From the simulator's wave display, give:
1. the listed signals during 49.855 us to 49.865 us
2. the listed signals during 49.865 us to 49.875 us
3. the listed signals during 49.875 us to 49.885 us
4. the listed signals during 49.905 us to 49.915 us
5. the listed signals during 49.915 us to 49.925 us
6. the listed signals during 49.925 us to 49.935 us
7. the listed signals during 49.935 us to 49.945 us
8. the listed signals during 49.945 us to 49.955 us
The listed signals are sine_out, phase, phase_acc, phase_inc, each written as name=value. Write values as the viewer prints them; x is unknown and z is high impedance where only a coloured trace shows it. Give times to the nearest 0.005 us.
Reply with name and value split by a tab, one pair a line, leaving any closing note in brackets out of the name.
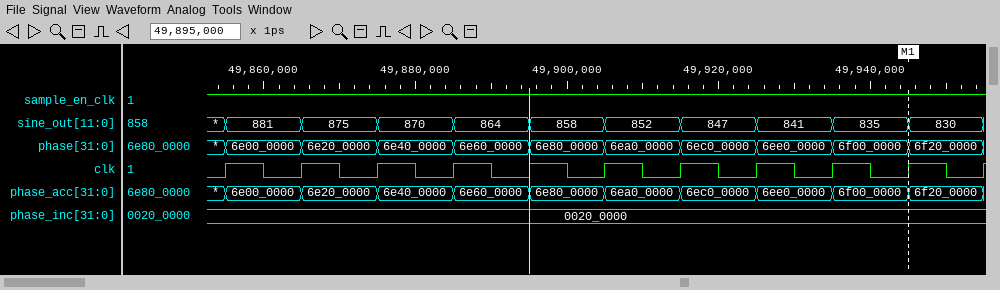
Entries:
the listed signals during 49.855 us to 49.865 us	sine_out=881, phase=6e00_0000, phase_acc=6e00_0000, phase_inc=0020_0000
the listed signals during 49.865 us to 49.875 us	sine_out=875, phase=6e20_0000, phase_acc=6e20_0000, phase_inc=0020_0000
the listed signals during 49.875 us to 49.885 us	sine_out=870, phase=6e40_0000, phase_acc=6e40_0000, phase_inc=0020_0000
the listed signals during 49.905 us to 49.915 us	sine_out=852, phase=6ea0_0000, phase_acc=6ea0_0000, phase_inc=0020_0000
the listed signals during 49.915 us to 49.925 us	sine_out=847, phase=6ec0_0000, phase_acc=6ec0_0000, phase_inc=0020_0000
the listed signals during 49.925 us to 49.935 us	sine_out=841, phase=6ee0_0000, phase_acc=6ee0_0000, phase_inc=0020_0000
the listed signals during 49.935 us to 49.945 us	sine_out=835, phase=6f00_0000, phase_acc=6f00_0000, phase_inc=0020_0000
the listed signals during 49.945 us to 49.955 us	sine_out=830, phase=6f20_0000, phase_acc=6f20_0000, phase_inc=0020_0000
